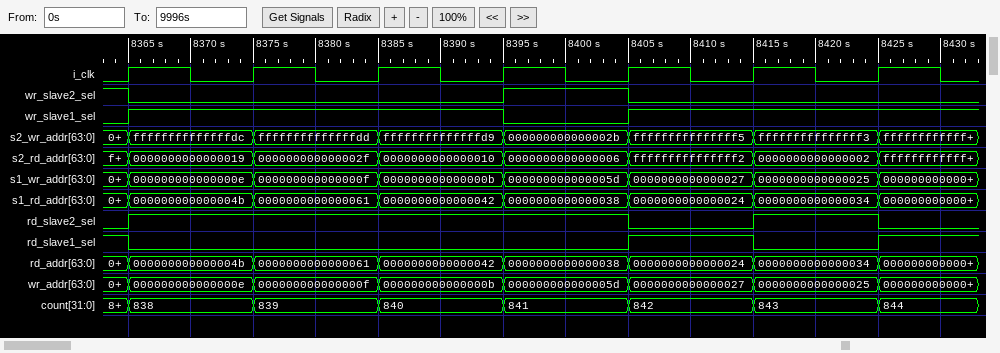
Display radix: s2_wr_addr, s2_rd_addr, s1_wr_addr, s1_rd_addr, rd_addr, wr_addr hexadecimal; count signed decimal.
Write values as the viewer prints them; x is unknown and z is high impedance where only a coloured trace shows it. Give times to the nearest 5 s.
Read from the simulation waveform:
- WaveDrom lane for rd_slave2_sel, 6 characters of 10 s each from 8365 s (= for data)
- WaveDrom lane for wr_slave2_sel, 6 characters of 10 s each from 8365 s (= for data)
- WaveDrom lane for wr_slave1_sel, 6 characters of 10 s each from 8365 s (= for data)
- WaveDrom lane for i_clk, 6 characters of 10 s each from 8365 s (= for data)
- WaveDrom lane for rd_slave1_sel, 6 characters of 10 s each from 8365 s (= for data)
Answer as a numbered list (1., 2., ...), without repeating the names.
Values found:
1. {name: 'rd_slave2_sel', wave: '1...01'}
2. {name: 'wr_slave2_sel', wave: '0..10.'}
3. {name: 'wr_slave1_sel', wave: '1..01.'}
4. {name: 'i_clk', wave: 'p.....'}
5. {name: 'rd_slave1_sel', wave: '0...10'}
